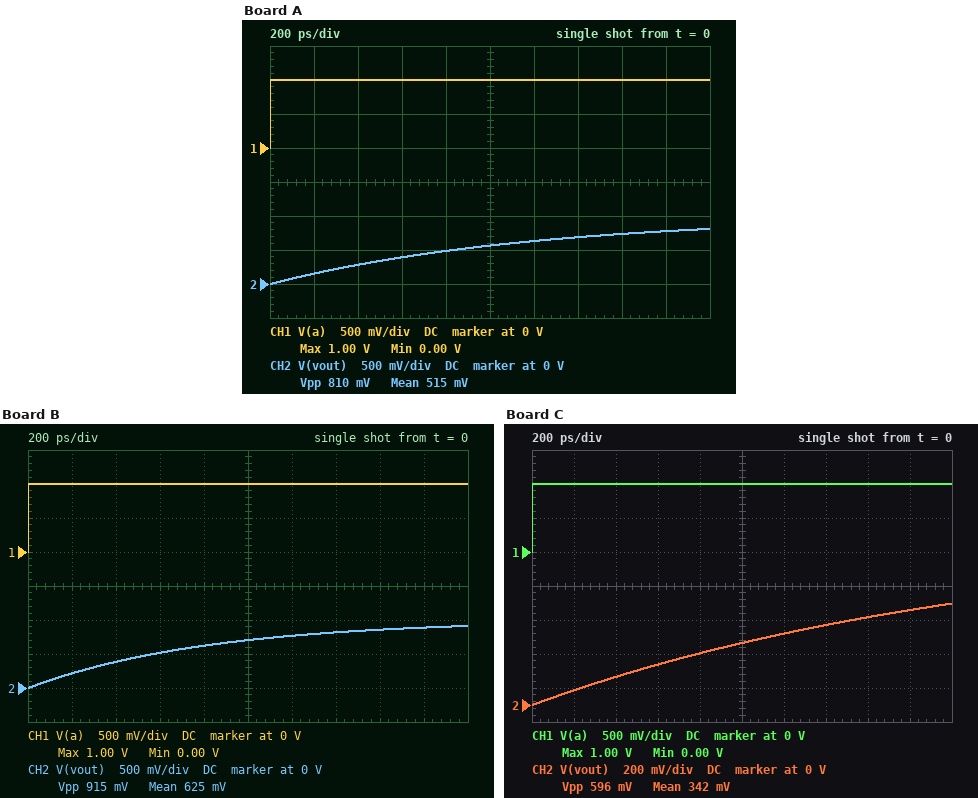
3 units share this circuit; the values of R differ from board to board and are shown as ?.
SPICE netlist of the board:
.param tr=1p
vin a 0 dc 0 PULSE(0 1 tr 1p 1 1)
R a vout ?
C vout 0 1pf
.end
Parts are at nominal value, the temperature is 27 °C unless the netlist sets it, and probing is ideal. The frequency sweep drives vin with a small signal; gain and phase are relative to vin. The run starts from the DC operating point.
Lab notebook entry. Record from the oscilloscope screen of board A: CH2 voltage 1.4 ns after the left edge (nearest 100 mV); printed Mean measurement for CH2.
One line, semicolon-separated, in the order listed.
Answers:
700 mV; 515 mV
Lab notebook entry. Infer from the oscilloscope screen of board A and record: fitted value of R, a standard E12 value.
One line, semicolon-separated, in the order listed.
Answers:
1.2 kΩ
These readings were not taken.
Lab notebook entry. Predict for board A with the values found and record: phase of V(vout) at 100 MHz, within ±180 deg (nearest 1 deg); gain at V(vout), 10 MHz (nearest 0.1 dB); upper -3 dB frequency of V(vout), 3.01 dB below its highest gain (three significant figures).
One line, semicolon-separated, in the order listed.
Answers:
-37 deg; 0 dB; 133 MHz
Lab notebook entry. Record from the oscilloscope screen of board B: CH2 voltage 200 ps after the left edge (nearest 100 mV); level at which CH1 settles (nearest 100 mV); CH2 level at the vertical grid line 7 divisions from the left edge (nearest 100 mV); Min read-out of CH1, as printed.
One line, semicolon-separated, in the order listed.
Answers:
200 mV; 1.0 V; 800 mV; 0.00 V
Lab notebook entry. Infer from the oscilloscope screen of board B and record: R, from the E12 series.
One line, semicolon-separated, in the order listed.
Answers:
820 Ω
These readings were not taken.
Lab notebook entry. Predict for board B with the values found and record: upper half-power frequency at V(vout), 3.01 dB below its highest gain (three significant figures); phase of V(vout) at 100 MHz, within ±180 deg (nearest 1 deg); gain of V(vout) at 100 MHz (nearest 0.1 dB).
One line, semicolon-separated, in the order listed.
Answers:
194 MHz; -27 deg; -1.0 dB
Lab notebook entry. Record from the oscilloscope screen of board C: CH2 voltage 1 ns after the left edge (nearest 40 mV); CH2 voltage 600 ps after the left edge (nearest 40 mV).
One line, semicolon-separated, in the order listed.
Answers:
360 mV; 240 mV
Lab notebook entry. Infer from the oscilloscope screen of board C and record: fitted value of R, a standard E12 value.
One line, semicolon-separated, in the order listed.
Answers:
2.2 kΩ
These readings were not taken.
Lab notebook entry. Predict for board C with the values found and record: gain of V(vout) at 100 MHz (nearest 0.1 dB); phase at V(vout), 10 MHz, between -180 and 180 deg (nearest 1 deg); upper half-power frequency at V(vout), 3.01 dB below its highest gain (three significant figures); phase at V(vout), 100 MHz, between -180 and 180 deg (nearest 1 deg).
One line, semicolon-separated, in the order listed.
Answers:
-4.6 dB; -8 deg; 72.3 MHz; -54 deg
